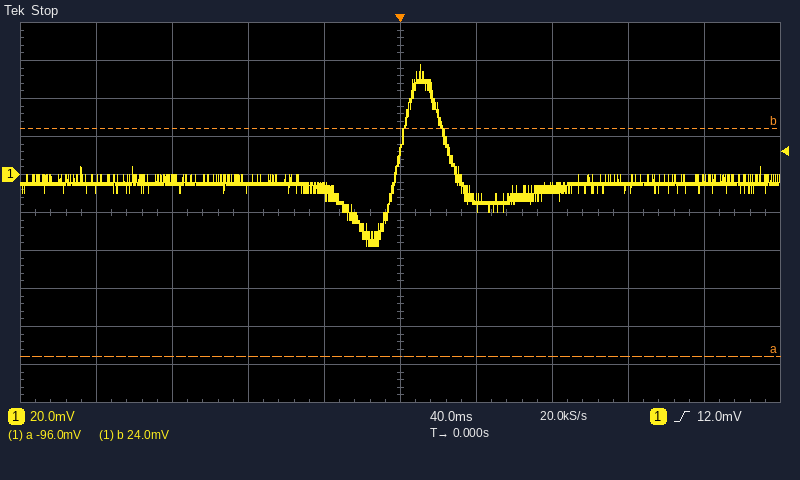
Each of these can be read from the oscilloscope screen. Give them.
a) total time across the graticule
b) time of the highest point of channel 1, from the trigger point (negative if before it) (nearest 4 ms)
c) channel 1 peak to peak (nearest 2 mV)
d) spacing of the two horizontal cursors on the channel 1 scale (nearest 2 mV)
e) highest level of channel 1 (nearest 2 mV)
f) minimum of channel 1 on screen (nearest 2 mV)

400 ms
+12 ms
96 mV
120 mV
58 mV
-38 mV
